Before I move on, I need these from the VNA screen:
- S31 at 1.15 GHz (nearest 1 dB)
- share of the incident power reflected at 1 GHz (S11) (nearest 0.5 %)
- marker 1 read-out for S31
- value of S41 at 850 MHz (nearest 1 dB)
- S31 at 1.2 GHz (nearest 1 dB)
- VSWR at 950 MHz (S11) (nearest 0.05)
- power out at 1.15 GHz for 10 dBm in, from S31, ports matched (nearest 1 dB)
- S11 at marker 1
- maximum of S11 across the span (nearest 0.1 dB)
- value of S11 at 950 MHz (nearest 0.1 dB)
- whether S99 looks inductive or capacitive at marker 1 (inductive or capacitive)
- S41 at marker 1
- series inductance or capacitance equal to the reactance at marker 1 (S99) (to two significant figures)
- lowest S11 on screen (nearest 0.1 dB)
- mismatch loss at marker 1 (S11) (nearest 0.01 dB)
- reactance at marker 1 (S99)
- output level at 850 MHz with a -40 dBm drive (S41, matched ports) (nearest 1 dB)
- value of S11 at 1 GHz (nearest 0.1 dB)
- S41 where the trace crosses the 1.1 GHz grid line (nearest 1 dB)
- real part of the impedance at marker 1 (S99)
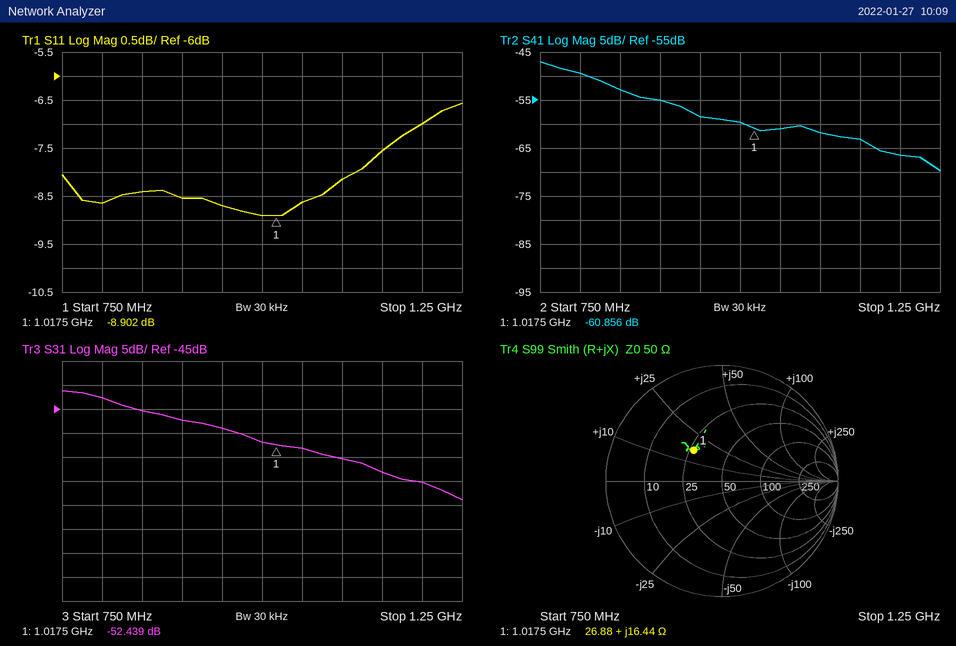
-58 dB
13.0 %
-52.439 dB
-53 dB
-60 dB
2.15
-48 dBm
-8.902 dB
-6.6 dB
-8.7 dB
inductive
-60.856 dB
2.6 nH
-8.9 dB
0.60 dB
+16.44 Ω
-93 dBm
-8.9 dB
-62 dB
26.88 Ω
